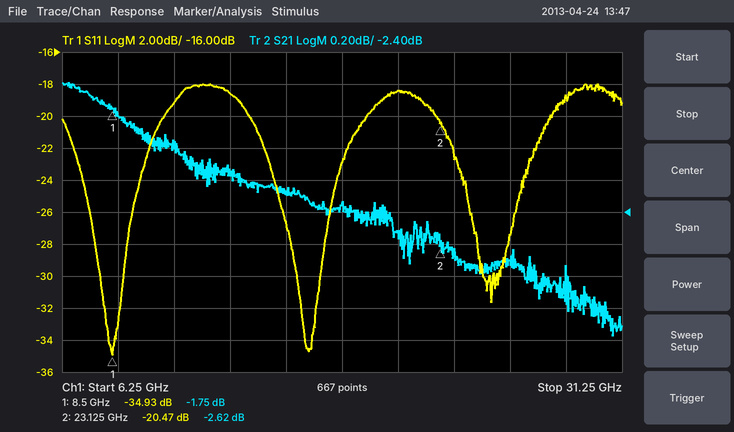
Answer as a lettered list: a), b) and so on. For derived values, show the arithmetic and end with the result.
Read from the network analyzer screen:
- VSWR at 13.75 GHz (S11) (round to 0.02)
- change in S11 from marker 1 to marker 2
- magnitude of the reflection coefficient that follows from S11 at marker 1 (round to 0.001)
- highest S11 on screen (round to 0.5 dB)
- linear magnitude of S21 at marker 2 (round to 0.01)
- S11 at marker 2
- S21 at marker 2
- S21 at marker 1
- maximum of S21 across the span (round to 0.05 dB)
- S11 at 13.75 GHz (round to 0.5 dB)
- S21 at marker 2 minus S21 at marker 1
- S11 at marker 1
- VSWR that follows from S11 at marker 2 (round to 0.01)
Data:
a) |Γ| = 10^(-18.5/20) = 0.1189; VSWR = (1 + 0.1189)/(1 − 0.1189) ≈ 1.27, so 1.26 to the nearest 0.02
b) -20.47 − (-34.93) = 14.46 dB
c) 10^(-34.93/20) ≈ 0.018
d) -18.0 dB
e) 10^(-2.62/20) ≈ 0.74
f) -20.47 dB
g) -2.62 dB
h) -1.75 dB
i) -1.60 dB
j) -18.5 dB
k) -2.62 − (-1.75) = -0.87 dB
l) -34.93 dB
m) (1 + 0.0947)/(1 − 0.0947) ≈ 1.21
